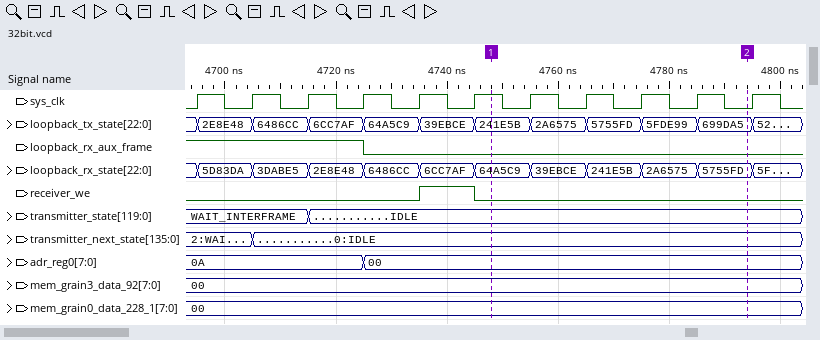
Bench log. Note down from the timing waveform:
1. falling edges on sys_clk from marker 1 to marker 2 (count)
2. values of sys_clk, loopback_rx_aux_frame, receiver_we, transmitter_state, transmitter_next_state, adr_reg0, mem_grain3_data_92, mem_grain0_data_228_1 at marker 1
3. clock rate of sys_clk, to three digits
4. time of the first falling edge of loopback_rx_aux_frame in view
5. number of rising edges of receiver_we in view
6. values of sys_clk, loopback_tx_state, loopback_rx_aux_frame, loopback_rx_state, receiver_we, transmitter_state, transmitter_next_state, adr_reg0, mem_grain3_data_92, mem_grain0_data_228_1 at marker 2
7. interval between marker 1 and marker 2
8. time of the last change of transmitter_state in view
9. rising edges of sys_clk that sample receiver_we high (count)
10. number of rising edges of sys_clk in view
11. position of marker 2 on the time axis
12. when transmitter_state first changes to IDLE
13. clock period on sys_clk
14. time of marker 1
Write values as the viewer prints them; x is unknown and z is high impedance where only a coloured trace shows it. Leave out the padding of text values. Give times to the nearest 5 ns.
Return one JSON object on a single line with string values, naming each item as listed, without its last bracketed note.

{"falling edges on sys_clk from marker 1 to marker 2": "5", "values of sys_clk, loopback_rx_aux_frame, receiver_we, transmitter_state, transmitter_next_state, adr_reg0, mem_grain3_data_92, mem_grain0_data_228_1 at marker 1": "sys_clk=1, loopback_rx_aux_frame=0, receiver_we=0, transmitter_state=IDLE, transmitter_next_state=0:IDLE, adr_reg0=00, mem_grain3_data_92=00, mem_grain0_data_228_1=00", "clock rate of sys_clk, to three digits": "100 MHz", "time of the first falling edge of loopback_rx_aux_frame in view": "4725 ns", "number of rising edges of receiver_we in view": "1", "values of sys_clk, loopback_tx_state, loopback_rx_aux_frame, loopback_rx_state, receiver_we, transmitter_state, transmitter_next_state, adr_reg0, mem_grain3_data_92, mem_grain0_data_228_1 at marker 2": "sys_clk=0, loopback_tx_state=699DA5, loopback_rx_aux_frame=0, loopback_rx_state=5755FD, receiver_we=0, transmitter_state=IDLE, transmitter_next_state=0:IDLE, adr_reg0=00, mem_grain3_data_92=00, mem_grain0_data_228_1=00", "interval between marker 1 and marker 2": "45 ns", "time of the last change of transmitter_state in view": "4715 ns", "rising edges of sys_clk that sample receiver_we high": "1", "number of rising edges of sys_clk in view": "11", "position of marker 2 on the time axis": "4795 ns", "when transmitter_state first changes to IDLE": "4715 ns", "clock period on sys_clk": "10 ns", "time of marker 1": "4750 ns"}
